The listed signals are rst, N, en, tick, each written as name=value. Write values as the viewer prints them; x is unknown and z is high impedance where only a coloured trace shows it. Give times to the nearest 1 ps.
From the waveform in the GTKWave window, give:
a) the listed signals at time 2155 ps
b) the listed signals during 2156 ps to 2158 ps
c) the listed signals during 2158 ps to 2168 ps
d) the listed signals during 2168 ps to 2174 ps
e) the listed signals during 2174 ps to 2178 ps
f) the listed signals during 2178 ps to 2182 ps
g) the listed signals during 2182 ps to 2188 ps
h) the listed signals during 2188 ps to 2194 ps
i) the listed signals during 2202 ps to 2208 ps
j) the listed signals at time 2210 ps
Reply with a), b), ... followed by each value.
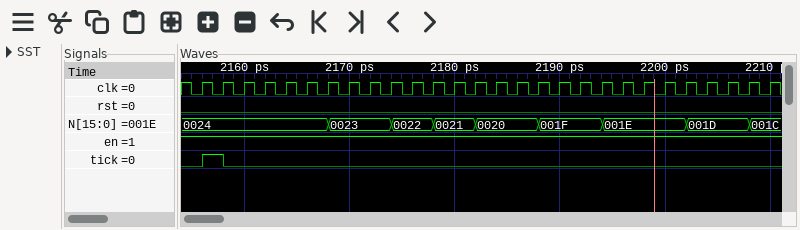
a) rst=0, N=0024, en=1, tick=0
b) rst=0, N=0024, en=1, tick=1
c) rst=0, N=0024, en=1, tick=0
d) rst=0, N=0023, en=1, tick=0
e) rst=0, N=0022, en=1, tick=0
f) rst=0, N=0021, en=1, tick=0
g) rst=0, N=0020, en=1, tick=0
h) rst=0, N=001F, en=1, tick=0
i) rst=0, N=001D, en=1, tick=0
j) rst=0, N=001C, en=1, tick=0
